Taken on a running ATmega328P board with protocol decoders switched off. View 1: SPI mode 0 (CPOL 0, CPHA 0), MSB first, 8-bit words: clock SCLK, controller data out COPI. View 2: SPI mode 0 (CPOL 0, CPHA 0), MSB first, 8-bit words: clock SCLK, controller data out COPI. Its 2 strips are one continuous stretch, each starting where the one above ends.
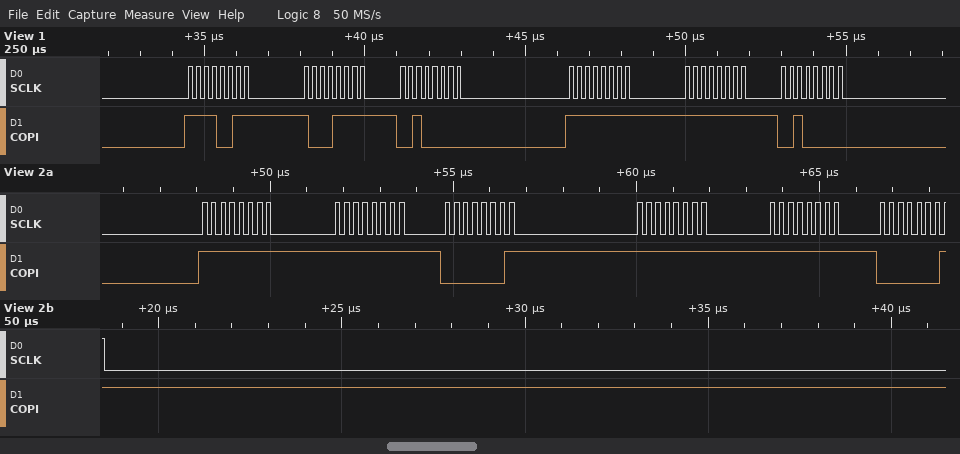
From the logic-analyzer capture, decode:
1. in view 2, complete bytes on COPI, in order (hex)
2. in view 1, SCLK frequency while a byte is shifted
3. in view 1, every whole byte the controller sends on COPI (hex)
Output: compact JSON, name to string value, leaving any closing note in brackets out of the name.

{"in view 2, complete bytes on COPI, in order": "FF FF 01 FF FF 01", "in view 1, SCLK frequency while a byte is shifted": "4 MHz", "in view 1, every whole byte the controller sends on COPI": "F3 8F 20 FF FF 20"}
